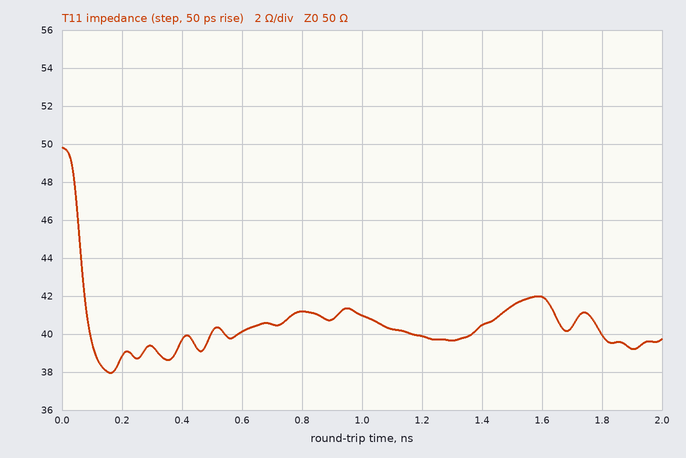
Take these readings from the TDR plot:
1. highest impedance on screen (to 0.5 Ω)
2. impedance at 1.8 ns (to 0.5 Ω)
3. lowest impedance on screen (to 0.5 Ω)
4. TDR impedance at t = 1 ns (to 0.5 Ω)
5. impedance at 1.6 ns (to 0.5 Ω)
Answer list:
50.0 Ω
40.0 Ω
38.0 Ω
41.0 Ω
42.0 Ω
